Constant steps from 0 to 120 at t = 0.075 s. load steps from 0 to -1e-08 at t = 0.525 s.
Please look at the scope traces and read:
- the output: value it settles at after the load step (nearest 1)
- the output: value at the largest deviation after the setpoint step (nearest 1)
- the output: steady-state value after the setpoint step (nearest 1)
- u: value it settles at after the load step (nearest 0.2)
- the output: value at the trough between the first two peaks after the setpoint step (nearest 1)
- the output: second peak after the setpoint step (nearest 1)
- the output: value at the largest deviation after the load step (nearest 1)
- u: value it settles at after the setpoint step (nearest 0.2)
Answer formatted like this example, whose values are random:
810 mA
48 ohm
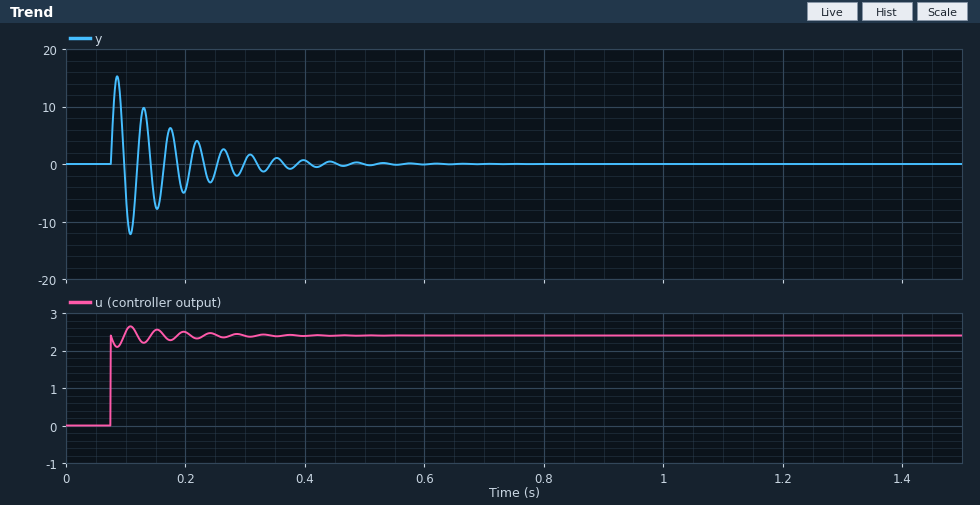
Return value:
0
15
0
2.4
-12
10
0
2.4
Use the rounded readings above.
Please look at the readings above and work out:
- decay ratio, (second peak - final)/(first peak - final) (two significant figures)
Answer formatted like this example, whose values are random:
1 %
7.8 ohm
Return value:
0.67
